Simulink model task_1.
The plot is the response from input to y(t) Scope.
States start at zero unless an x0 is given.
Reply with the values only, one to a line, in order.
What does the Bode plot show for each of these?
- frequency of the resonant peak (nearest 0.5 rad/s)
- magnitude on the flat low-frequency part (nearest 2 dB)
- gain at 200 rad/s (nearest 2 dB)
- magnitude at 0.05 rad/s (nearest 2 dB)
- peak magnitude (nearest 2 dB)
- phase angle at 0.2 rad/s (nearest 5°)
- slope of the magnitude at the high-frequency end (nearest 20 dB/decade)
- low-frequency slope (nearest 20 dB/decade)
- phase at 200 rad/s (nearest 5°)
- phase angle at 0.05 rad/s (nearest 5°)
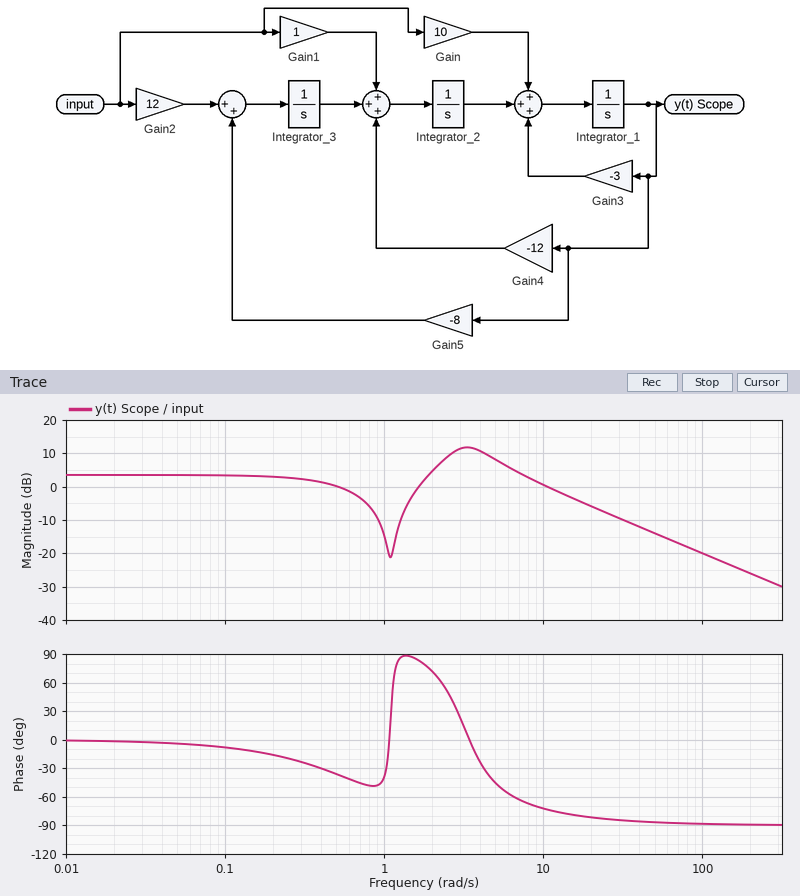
3.5 rad/s
4 dB
-26 dB
4 dB
12 dB
-15°
-20 dB/decade
0 dB/decade
-90°
-5°
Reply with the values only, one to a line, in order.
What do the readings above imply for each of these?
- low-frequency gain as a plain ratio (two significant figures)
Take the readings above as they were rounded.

1.6
